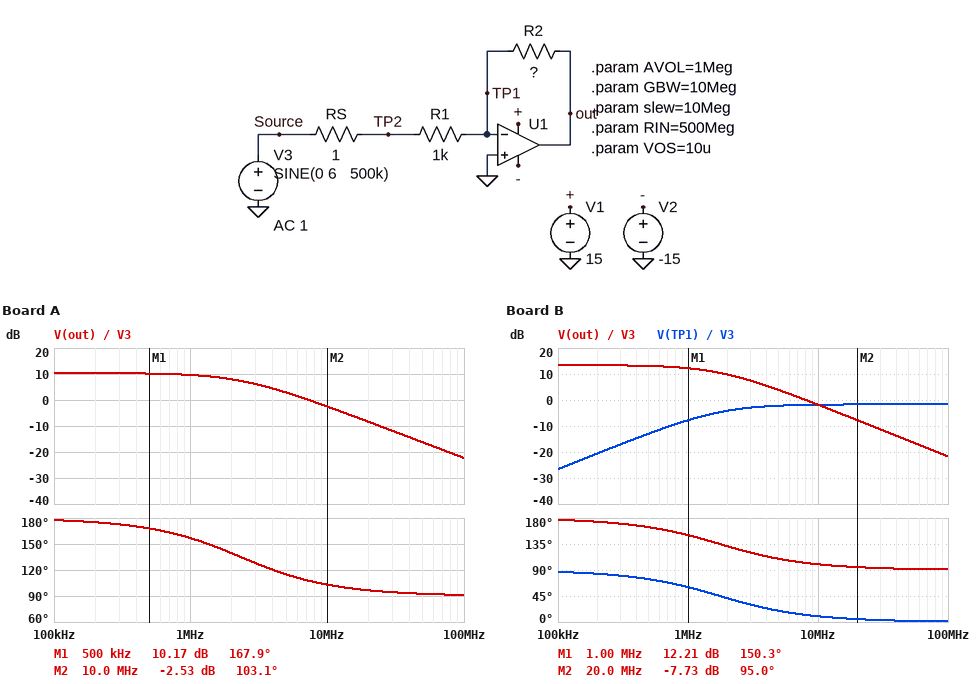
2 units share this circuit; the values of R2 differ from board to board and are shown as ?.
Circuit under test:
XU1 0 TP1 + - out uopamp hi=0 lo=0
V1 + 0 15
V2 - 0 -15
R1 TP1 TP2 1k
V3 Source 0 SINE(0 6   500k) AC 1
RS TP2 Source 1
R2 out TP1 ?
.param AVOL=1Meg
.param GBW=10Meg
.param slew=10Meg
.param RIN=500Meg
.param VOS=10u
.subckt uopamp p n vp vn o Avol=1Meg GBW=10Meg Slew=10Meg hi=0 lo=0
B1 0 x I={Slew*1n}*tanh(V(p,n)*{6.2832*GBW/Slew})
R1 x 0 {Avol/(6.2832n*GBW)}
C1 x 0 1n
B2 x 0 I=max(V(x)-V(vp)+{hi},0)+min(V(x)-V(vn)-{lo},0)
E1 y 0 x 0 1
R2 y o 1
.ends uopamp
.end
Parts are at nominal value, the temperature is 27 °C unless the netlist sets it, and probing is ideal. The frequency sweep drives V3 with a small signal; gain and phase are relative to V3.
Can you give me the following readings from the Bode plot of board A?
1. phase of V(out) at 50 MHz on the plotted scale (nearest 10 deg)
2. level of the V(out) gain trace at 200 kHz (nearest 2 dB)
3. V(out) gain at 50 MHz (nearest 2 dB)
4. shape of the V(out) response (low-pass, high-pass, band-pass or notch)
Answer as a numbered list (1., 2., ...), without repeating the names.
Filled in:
1. 90 deg
2. 10 dB
3. -16 dB
4. low-pass
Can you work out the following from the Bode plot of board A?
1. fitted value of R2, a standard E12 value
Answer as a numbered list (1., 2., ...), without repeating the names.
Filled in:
1. 3.3 kΩ
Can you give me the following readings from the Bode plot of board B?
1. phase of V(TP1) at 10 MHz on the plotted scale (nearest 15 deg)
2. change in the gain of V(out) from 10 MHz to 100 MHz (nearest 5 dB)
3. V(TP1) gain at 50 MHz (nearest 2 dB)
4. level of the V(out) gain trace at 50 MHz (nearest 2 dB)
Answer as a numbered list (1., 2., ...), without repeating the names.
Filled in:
1. 15 deg
2. -20 dB
3. -2 dB
4. -16 dB
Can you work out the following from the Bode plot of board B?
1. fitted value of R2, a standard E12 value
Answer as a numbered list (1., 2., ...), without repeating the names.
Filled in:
1. 4.7 kΩ
